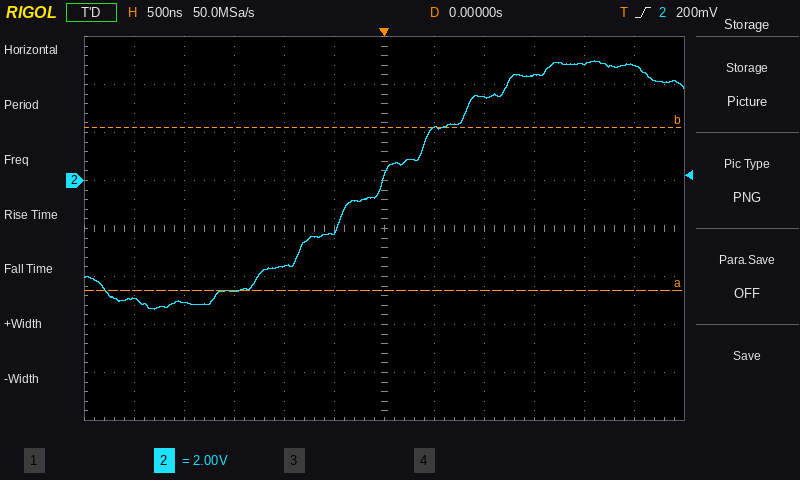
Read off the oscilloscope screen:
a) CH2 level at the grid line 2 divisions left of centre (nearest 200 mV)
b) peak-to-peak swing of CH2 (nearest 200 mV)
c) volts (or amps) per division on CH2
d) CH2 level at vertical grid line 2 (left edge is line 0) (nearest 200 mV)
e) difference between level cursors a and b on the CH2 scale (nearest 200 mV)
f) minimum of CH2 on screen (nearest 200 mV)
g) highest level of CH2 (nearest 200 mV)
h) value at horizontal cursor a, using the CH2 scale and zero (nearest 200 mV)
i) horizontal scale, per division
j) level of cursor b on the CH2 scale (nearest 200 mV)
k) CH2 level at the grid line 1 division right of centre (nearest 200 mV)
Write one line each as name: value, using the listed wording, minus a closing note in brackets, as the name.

CH2 level at the grid line 2 divisions left of centre: -3.6 V
peak-to-peak swing of CH2: 10.4 V
volts (or amps) per division on CH2: 2 V
CH2 level at vertical grid line 2 (left edge is line 0): -5.0 V
difference between level cursors a and b on the CH2 scale: 6.8 V
minimum of CH2 on screen: -5.4 V
highest level of CH2: 5.0 V
value at horizontal cursor a, using the CH2 scale and zero: -4.6 V
horizontal scale, per division: 500 ns
level of cursor b on the CH2 scale: 2.2 V
CH2 level at the grid line 1 division right of centre: 2.2 V
